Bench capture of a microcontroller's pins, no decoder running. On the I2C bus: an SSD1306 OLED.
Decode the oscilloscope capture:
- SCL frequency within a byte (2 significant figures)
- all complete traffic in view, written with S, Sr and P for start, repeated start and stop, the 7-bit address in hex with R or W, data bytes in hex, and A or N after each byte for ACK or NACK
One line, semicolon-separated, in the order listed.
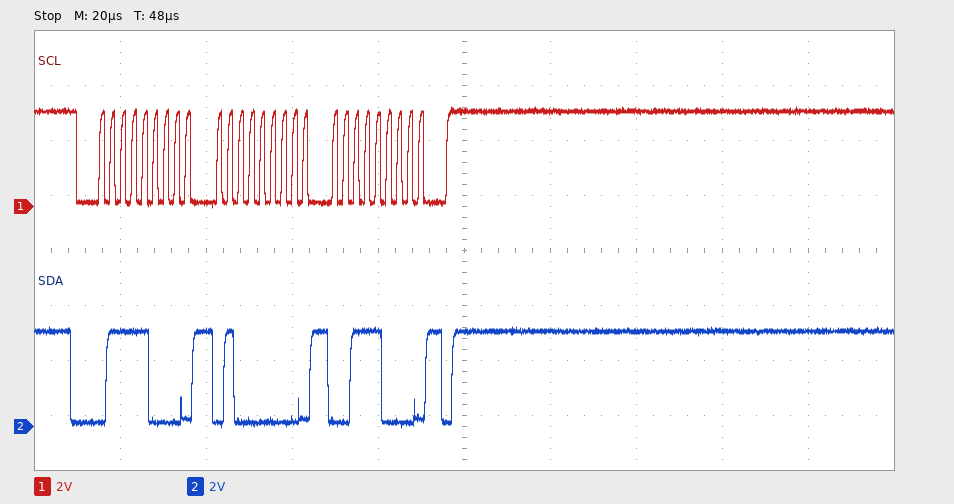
400 kHz; S 3CW A 40 A 38 A P
